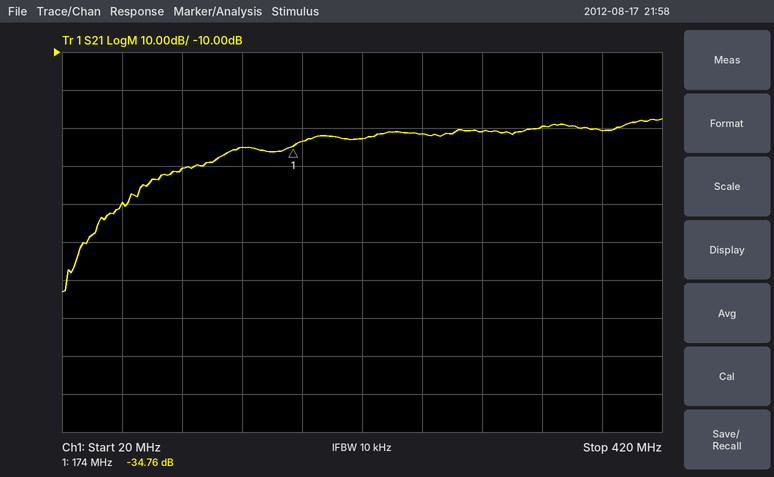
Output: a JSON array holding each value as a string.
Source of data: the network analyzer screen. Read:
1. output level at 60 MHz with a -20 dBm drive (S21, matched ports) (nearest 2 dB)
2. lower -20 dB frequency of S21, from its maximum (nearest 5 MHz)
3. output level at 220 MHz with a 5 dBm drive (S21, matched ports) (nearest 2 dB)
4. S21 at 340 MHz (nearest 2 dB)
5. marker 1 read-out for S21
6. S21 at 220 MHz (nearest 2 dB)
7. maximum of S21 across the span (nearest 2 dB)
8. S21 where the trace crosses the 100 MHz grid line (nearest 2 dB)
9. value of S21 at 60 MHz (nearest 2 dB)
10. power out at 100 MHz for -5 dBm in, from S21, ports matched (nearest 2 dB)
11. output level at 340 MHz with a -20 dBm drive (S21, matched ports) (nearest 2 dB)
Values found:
["-70 dBm", "70 MHz", "-28 dBm", "-30 dB", "-34.76 dB", "-32 dB", "-28 dB", "-40 dB", "-50 dB", "-46 dBm", "-50 dBm"]
